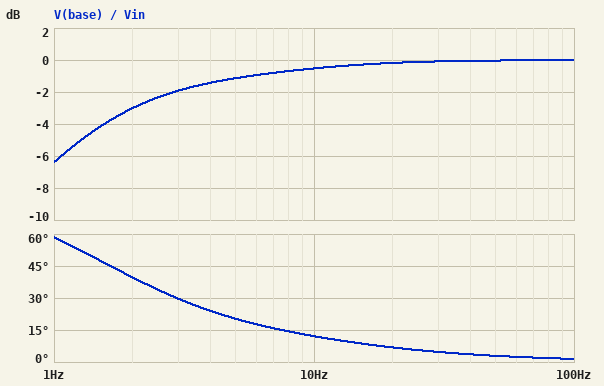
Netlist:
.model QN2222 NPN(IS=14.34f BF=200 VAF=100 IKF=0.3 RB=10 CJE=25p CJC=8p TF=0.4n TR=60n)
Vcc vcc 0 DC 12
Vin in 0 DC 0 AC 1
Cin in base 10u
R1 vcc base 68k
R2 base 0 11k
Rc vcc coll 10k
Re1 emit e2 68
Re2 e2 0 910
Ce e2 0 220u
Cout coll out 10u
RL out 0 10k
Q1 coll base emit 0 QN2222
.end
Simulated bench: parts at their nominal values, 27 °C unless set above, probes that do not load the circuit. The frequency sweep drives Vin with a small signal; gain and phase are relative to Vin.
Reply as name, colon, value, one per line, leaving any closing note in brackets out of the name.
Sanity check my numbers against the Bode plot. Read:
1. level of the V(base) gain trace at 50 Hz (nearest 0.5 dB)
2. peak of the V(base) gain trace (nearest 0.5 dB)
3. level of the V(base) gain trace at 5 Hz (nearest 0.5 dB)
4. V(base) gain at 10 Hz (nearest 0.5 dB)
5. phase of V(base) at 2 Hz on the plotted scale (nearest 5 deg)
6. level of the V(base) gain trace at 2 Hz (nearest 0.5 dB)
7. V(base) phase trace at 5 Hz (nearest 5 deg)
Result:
level of the V(base) gain trace at 50 Hz: 0 dB
peak of the V(base) gain trace: 0 dB
level of the V(base) gain trace at 5 Hz: -1.0 dB
V(base) gain at 10 Hz: -0.5 dB
phase of V(base) at 2 Hz on the plotted scale: 40 deg
level of the V(base) gain trace at 2 Hz: -3.0 dB
V(base) phase trace at 5 Hz: 20 deg
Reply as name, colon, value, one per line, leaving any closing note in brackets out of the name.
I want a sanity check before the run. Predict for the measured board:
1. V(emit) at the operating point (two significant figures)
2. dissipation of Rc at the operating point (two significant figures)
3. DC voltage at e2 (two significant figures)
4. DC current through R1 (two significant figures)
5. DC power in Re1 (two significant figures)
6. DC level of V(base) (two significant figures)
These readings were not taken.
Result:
V(emit) at the operating point: 980 mV
dissipation of Rc at the operating point: 9.9 mW
DC voltage at e2: 910 mV
DC current through R1: 150 µA
DC power in Re1: 68 µW
DC level of V(base): 1.6 V
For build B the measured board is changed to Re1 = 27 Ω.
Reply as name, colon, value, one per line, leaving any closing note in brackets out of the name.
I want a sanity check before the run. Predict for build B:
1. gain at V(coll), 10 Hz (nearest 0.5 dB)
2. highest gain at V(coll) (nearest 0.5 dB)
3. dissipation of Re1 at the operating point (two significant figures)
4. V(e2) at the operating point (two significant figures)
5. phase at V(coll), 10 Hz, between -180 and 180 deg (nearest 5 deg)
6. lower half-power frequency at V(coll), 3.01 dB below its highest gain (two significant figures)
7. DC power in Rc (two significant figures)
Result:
gain at V(coll), 10 Hz: 34.0 dB
highest gain at V(coll): 39.5 dB
dissipation of Re1 at the operating point: 29 µW
V(e2) at the operating point: 950 mV
phase at V(coll), 10 Hz, between -180 and 180 deg: -120 deg
lower half-power frequency at V(coll), 3.01 dB below its highest gain: 16 Hz
DC power in Rc: 11 mW
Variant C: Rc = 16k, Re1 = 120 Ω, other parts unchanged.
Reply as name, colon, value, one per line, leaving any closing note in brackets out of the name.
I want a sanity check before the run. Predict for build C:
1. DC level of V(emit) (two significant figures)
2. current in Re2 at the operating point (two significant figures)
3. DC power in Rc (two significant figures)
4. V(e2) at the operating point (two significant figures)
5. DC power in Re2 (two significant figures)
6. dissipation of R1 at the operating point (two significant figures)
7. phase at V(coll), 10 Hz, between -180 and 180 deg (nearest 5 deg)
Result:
DC level of V(emit): 750 mV
current in Re2 at the operating point: 730 µA
DC power in Rc: 7.8 mW
V(e2) at the operating point: 660 mV
DC power in Re2: 480 µW
dissipation of R1 at the operating point: 1.7 mW
phase at V(coll), 10 Hz, between -180 and 180 deg: -90 deg
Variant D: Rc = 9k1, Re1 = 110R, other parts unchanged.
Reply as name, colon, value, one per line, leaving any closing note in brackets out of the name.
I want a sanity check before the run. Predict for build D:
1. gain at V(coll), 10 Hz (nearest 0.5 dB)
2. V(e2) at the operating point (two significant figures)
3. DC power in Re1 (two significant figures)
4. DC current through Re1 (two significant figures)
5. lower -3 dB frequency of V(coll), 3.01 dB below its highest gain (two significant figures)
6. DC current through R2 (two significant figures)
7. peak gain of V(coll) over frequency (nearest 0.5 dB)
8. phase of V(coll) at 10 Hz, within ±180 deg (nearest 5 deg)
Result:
gain at V(coll), 10 Hz: 29.0 dB
V(e2) at the operating point: 880 mV
DC power in Re1: 100 µW
DC current through Re1: 960 µA
lower -3 dB frequency of V(coll), 3.01 dB below its highest gain: 6.7 Hz
DC current through R2: 150 µA
peak gain of V(coll) over frequency: 30.5 dB
phase of V(coll) at 10 Hz, within ±180 deg: -145 deg
